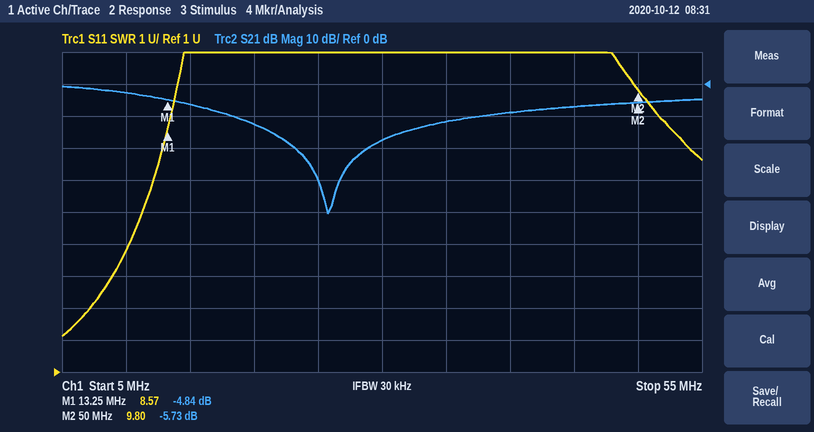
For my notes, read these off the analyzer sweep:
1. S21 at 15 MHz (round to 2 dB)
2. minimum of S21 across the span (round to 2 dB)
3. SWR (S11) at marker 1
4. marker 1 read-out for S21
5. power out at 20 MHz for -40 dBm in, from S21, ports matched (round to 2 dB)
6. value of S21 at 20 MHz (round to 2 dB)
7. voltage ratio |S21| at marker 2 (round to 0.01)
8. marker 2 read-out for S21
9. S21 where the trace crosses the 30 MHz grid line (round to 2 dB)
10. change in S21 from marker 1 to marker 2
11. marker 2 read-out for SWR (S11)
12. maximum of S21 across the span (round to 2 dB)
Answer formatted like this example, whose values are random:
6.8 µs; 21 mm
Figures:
-6 dB; -40 dB; 8.57; -4.84 dB; -52 dBm; -12 dB; 0.52; -5.73 dB; -18 dB; -0.89 dB; 9.80; 0 dB
